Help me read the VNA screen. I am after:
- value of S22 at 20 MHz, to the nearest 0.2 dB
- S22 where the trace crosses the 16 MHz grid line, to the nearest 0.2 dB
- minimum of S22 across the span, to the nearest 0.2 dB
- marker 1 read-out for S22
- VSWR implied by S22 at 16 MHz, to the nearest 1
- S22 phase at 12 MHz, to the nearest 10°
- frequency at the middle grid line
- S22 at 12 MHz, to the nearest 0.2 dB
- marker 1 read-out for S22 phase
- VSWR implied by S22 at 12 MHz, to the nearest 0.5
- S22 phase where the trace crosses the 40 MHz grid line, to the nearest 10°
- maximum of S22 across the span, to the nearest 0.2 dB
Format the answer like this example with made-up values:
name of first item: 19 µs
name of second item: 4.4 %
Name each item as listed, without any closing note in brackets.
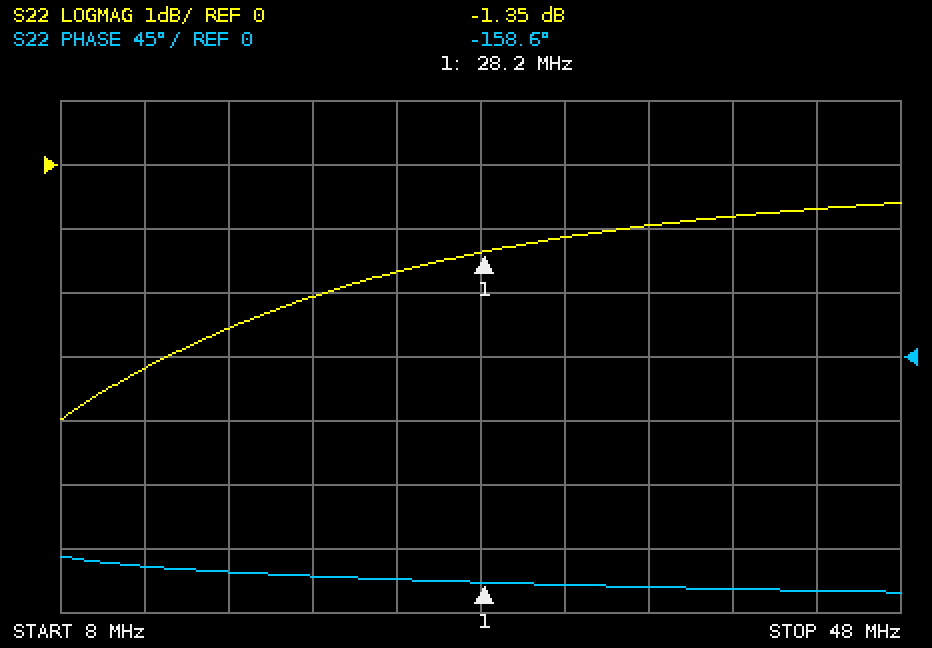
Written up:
value of S22 at 20 MHz, to the nearest 0.2 dB: -2.0 dB
S22 where the trace crosses the 16 MHz grid line, to the nearest 0.2 dB: -2.6 dB
minimum of S22 across the span, to the nearest 0.2 dB: -4.0 dB
marker 1 read-out for S22: -1.35 dB
VSWR implied by S22 at 16 MHz, to the nearest 1: 7
S22 phase at 12 MHz, to the nearest 10°: -150°
frequency at the middle grid line: 28 MHz
S22 at 12 MHz, to the nearest 0.2 dB: -3.2 dB
marker 1 read-out for S22 phase: -158.6°
VSWR implied by S22 at 12 MHz, to the nearest 0.5: 5.5
S22 phase where the trace crosses the 40 MHz grid line, to the nearest 10°: -160°
maximum of S22 across the span, to the nearest 0.2 dB: -0.6 dB
